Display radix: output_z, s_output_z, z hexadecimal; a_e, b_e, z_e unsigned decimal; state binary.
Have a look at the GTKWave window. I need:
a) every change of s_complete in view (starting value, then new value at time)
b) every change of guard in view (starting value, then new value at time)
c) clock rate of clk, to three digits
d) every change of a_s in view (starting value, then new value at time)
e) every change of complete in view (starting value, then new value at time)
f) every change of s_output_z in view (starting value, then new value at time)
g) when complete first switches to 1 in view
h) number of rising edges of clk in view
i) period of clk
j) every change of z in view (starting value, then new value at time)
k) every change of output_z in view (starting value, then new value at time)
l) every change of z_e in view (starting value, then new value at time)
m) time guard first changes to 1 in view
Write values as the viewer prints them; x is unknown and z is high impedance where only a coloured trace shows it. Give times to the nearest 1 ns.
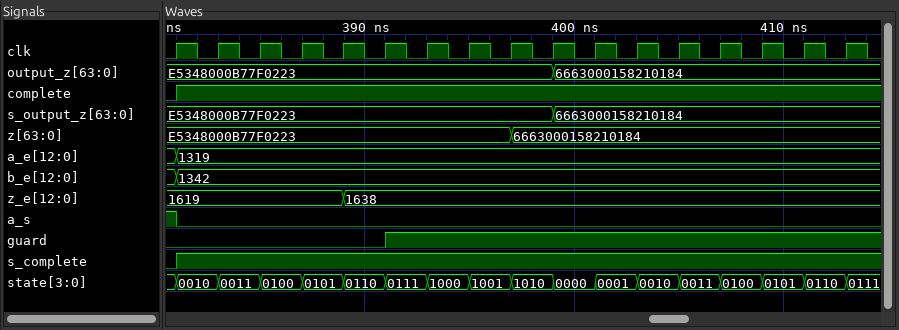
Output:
0, 1 at 381 ns
0, 1 at 391 ns
500 MHz
1, 0 at 381 ns
0, 1 at 381 ns
E5348000B77F0223, 6663000158210184 at 399 ns
381 ns
17
2 ns
E5348000B77F0223, 6663000158210184 at 397 ns
E5348000B77F0223, 6663000158210184 at 399 ns
1619, 1638 at 389 ns
391 ns
